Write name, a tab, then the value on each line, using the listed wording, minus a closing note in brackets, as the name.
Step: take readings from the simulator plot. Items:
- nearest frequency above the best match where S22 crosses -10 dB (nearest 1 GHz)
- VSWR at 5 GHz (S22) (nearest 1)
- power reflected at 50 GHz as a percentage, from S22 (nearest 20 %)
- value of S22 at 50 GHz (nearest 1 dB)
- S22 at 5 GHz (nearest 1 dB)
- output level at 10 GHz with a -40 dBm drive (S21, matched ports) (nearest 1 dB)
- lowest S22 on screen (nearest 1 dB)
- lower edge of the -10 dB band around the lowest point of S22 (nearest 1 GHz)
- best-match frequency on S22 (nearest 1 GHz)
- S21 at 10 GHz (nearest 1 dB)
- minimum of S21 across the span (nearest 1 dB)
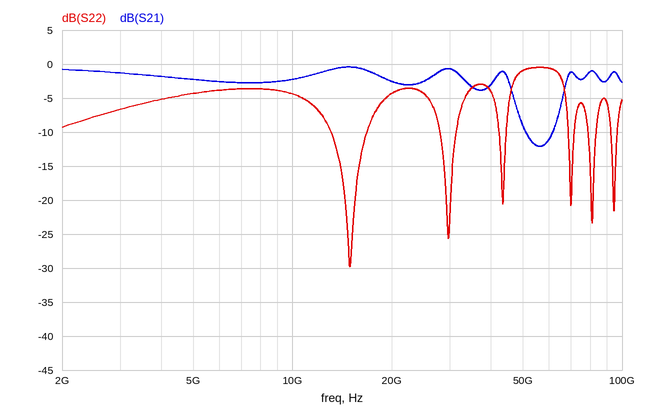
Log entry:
nearest frequency above the best match where S22 crosses -10 dB	17 GHz
VSWR at 5 GHz (S22)	4
power reflected at 50 GHz as a percentage, from S22	80 %
value of S22 at 50 GHz	-1 dB
S22 at 5 GHz	-4 dB
output level at 10 GHz with a -40 dBm drive (S21, matched ports)	-42 dBm
lowest S22 on screen	-30 dB
lower edge of the -10 dB band around the lowest point of S22	13 GHz
best-match frequency on S22	15 GHz
S21 at 10 GHz	-2 dB
minimum of S21 across the span	-12 dB
